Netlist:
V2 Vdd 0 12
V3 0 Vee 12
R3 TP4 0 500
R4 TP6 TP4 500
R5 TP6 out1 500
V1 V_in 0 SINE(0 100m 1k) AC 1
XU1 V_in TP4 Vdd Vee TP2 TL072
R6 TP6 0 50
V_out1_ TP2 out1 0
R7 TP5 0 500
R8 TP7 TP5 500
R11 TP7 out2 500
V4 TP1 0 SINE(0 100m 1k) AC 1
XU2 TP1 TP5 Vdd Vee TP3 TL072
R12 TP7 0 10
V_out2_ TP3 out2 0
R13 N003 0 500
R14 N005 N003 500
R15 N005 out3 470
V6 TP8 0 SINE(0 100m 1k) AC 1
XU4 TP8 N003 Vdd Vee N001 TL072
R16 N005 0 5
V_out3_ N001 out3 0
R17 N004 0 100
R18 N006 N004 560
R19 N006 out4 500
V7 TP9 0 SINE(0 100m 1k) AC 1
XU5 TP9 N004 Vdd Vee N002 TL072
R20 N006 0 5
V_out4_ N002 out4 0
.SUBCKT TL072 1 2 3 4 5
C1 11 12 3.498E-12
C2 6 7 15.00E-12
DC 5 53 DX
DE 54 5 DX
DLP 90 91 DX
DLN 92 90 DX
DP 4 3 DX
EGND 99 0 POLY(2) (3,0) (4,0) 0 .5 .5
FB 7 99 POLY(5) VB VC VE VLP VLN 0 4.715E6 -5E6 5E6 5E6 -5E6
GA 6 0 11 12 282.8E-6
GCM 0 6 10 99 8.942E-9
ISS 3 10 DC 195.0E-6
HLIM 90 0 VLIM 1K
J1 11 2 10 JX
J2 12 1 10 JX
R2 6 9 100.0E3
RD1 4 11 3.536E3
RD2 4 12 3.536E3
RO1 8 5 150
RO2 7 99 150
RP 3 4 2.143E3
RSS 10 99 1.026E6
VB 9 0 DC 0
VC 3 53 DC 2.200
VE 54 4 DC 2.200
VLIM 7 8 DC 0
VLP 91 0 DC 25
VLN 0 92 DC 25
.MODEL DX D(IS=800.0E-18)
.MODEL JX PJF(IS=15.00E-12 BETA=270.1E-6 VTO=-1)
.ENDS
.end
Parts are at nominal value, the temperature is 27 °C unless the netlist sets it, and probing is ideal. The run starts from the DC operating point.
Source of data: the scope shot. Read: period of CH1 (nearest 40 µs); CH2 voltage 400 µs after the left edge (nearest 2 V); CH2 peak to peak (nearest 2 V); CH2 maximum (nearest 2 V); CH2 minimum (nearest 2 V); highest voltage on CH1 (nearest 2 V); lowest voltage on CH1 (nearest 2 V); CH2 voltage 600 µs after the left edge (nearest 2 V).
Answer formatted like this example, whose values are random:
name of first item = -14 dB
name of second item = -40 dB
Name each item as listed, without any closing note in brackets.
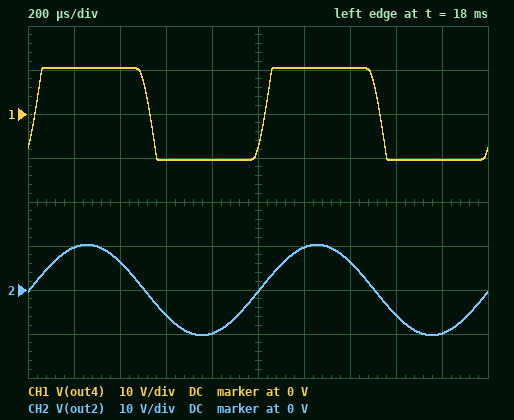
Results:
period of CH1 = 1.00 ms
CH2 voltage 400 µs after the left edge = 6 V
CH2 peak to peak = 20 V
CH2 maximum = 10 V
CH2 minimum = -10 V
highest voltage on CH1 = 10 V
lowest voltage on CH1 = -10 V
CH2 voltage 600 µs after the left edge = -6 V
